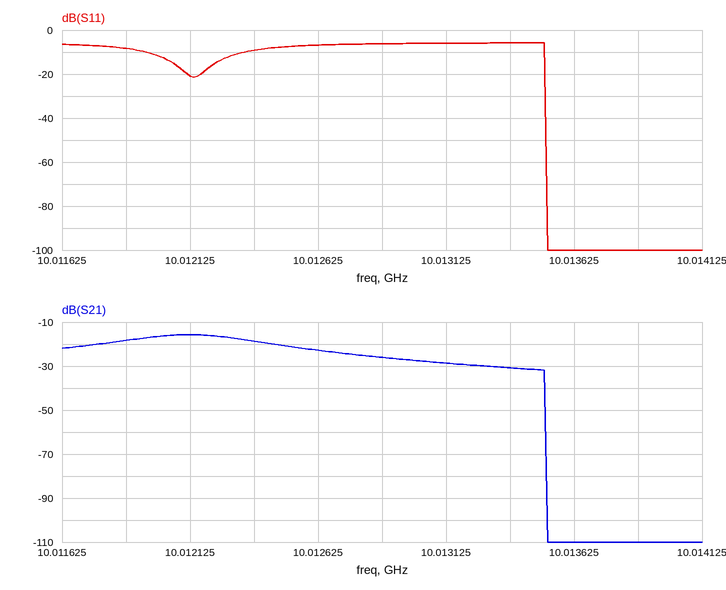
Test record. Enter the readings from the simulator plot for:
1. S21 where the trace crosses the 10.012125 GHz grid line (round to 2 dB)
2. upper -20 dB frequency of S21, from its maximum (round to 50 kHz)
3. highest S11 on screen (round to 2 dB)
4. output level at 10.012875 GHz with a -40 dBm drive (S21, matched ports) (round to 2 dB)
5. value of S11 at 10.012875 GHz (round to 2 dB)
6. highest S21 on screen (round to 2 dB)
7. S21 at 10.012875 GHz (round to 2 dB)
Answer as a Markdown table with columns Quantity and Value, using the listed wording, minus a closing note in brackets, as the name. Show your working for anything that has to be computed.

| Quantity | Value |
|---|---|
| S21 where the trace crosses the 10.012125 GHz grid line | -16 dB |
| upper -20 dB frequency of S21, from its maximum | 10.01350 GHz |
| highest S11 on screen | -6 dB |
| output level at 10.012875 GHz with a -40 dBm drive (S21, matched ports) | -40 dBm + (-26 dB) = -66 dBm |
| value of S11 at 10.012875 GHz | -6 dB |
| highest S21 on screen | -16 dB |
| S21 at 10.012875 GHz | -26 dB |
